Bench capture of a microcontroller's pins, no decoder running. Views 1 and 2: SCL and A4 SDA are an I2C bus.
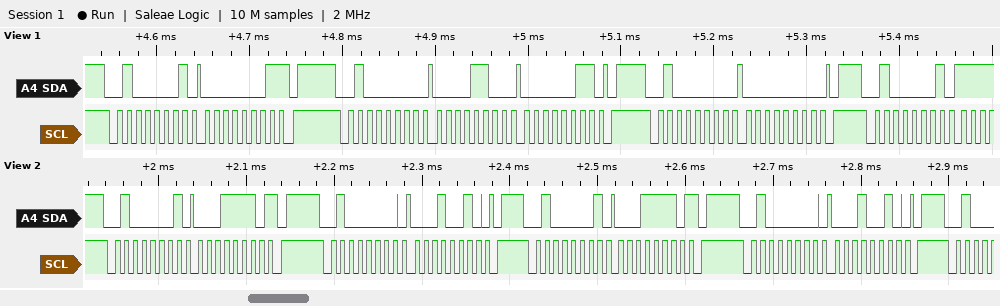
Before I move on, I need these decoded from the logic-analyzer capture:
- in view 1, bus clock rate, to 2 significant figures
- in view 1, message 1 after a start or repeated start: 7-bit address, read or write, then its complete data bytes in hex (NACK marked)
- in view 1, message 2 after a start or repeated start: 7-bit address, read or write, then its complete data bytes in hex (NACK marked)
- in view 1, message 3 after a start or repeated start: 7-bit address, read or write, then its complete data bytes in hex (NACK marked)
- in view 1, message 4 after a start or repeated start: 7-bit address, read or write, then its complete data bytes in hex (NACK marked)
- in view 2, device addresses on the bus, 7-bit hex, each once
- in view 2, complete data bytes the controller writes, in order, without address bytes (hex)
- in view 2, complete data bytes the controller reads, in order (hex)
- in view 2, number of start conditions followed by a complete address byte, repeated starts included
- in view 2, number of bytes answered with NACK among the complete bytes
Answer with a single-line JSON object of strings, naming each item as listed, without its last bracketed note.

{"in view 1, bus clock rate, to 2 significant figures": "100 kHz", "in view 1, message 1 after a start or repeated start: 7-bit address, read or write, then its complete data bytes in hex": "0x20 read: 01 NACK", "in view 1, message 2 after a start or repeated start: 7-bit address, read or write, then its complete data bytes in hex": "0x20 write: 0C 03", "in view 1, message 3 after a start or repeated start: 7-bit address, read or write, then its complete data bytes in hex": "0x20 write: 00", "in view 1, message 4 after a start or repeated start: 7-bit address, read or write, then its complete data bytes in hex": "0x20 read", "in view 2, device addresses on the bus, 7-bit hex, each once": "0x20", "in view 2, complete data bytes the controller writes, in order, without address bytes": "12 12", "in view 2, complete data bytes the controller reads, in order": "1E 1E", "in view 2, number of start conditions followed by a complete address byte, repeated starts included": "4", "in view 2, number of bytes answered with NACK among the complete bytes": "2"}
